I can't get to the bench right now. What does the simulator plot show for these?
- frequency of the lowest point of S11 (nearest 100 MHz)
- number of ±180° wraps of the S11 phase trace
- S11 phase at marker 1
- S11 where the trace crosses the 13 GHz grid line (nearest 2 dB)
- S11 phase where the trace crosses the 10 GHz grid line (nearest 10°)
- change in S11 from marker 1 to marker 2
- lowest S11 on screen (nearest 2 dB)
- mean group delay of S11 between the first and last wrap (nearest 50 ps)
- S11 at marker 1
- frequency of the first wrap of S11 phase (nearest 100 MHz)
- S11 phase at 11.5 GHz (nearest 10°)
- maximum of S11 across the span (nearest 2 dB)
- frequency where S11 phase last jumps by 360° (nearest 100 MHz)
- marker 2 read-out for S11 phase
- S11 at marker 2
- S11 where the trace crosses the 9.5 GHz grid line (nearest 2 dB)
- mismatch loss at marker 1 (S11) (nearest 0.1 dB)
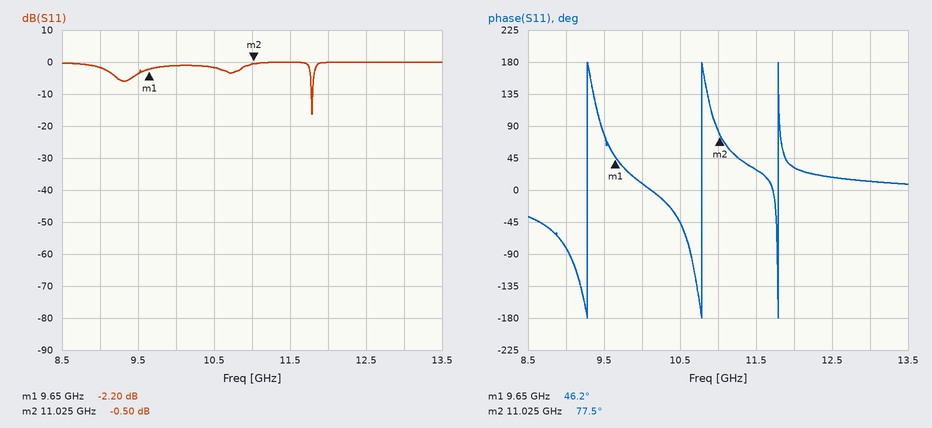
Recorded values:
11.8 GHz
3
46.2°
0 dB
10°
1.70 dB
-16 dB
800 ps
-2.20 dB
9.3 GHz
30°
0 dB
11.8 GHz
77.5°
-0.50 dB
-4 dB
4.0 dB
